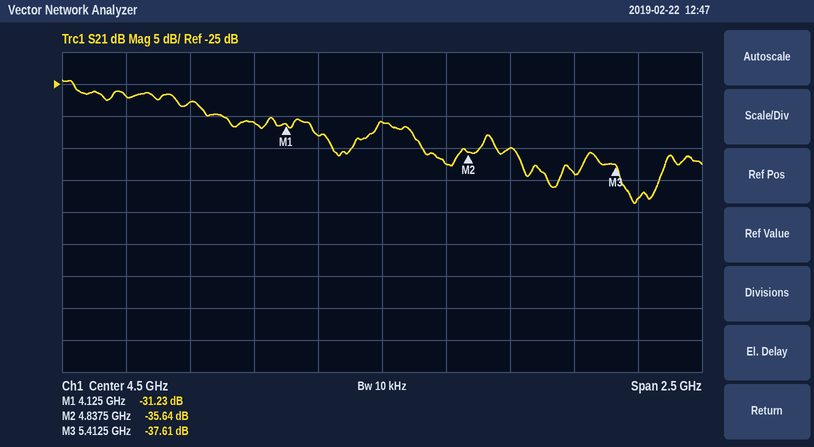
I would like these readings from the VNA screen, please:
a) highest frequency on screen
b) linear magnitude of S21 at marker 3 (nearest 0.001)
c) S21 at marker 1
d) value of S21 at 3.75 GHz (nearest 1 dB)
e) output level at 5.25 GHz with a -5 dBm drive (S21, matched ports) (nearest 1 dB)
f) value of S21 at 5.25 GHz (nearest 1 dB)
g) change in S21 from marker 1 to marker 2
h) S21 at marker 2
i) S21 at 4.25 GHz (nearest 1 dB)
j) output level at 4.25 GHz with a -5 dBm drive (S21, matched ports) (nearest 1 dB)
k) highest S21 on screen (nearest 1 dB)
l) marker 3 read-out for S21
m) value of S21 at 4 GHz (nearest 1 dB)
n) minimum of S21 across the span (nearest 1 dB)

5.75 GHz
0.013
-31.23 dB
-28 dB
-44 dBm
-39 dB
-4.41 dB
-35.64 dB
-33 dB
-38 dBm
-24 dB
-37.61 dB
-31 dB
-44 dB
